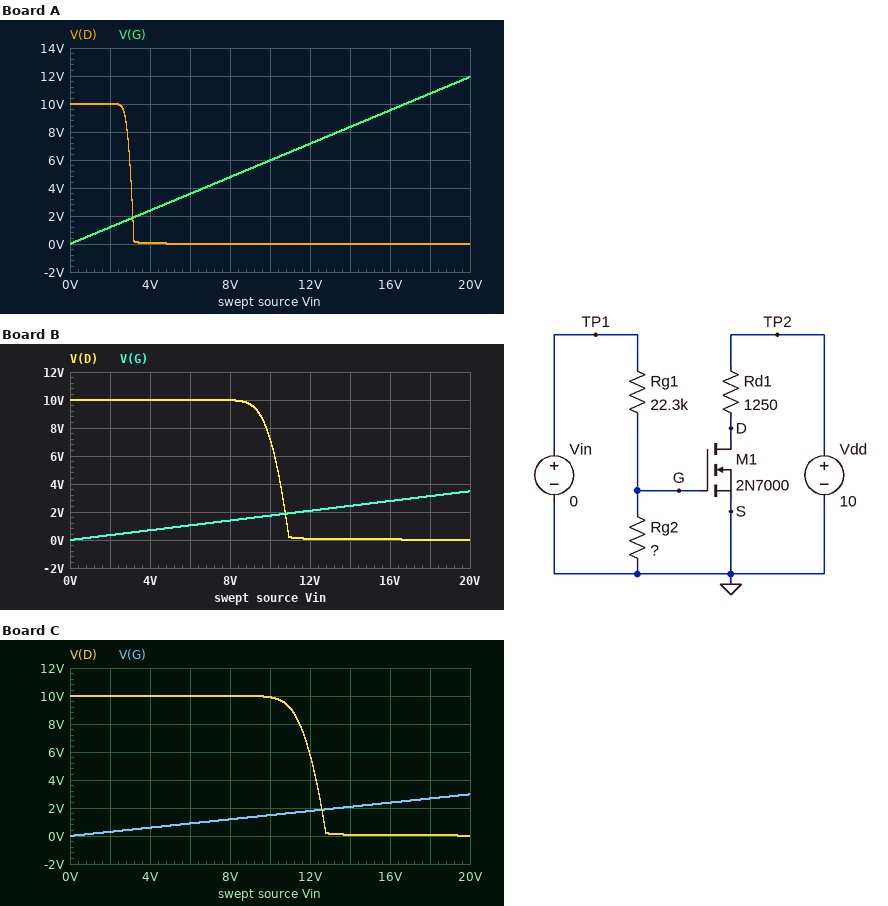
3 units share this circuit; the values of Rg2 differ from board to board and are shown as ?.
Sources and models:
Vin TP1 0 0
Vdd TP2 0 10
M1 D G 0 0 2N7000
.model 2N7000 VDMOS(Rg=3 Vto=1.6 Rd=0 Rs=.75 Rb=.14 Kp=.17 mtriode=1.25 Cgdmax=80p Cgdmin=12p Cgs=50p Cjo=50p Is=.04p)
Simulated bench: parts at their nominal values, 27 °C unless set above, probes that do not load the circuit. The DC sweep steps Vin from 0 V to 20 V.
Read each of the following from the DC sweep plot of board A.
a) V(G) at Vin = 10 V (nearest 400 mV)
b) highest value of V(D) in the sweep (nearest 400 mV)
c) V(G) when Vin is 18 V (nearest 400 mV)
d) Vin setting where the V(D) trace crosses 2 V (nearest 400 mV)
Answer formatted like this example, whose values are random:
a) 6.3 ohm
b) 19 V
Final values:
a) 6.0 V
b) 10.0 V
c) 10.8 V
d) 3.2 V
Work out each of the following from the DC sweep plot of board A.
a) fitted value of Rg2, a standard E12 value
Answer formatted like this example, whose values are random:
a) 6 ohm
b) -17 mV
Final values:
a) 33 kΩ
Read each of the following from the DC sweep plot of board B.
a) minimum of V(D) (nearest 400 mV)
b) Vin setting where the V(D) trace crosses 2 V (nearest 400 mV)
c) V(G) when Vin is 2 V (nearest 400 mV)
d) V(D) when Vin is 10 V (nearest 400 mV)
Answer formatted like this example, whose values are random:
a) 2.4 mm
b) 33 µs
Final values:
a) 0 V
b) 10.8 V
c) 400 mV
d) 7.2 V
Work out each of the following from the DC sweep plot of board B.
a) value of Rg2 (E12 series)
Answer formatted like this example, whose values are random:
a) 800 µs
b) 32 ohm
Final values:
a) 4.7 kΩ
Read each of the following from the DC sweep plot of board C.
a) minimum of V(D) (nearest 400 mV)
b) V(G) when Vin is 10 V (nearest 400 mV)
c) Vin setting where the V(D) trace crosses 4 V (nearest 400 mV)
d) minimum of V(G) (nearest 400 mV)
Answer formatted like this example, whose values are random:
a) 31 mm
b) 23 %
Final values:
a) 0 V
b) 1.6 V
c) 12.4 V
d) 0 V
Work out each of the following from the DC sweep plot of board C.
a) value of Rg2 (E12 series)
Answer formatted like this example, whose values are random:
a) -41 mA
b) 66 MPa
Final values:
a) 3.9 kΩ
